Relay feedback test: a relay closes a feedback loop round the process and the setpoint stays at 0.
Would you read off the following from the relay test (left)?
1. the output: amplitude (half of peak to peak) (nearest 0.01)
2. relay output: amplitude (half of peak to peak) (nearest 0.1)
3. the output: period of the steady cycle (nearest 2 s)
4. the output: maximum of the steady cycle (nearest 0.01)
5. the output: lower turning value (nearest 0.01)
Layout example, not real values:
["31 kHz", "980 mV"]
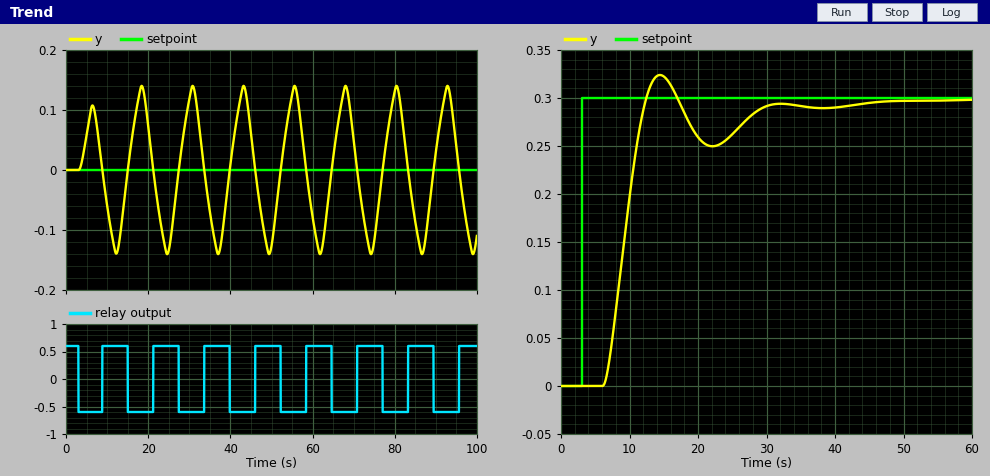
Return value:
["0.14", "0.6", "12 s", "0.14", "-0.14"]
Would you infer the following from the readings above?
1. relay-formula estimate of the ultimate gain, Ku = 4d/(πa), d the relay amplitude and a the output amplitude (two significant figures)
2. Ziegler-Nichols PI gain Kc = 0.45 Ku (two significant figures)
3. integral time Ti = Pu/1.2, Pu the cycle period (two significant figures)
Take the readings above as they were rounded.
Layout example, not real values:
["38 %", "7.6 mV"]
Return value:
["5.5", "2.5", "10 s"]
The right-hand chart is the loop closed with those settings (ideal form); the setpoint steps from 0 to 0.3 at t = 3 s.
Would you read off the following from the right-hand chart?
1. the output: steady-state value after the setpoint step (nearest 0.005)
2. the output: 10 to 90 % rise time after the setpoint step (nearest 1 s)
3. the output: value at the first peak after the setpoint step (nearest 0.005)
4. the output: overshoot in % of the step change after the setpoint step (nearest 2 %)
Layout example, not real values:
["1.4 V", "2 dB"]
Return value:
["0.300", "4 s", "0.325", "8 %"]
